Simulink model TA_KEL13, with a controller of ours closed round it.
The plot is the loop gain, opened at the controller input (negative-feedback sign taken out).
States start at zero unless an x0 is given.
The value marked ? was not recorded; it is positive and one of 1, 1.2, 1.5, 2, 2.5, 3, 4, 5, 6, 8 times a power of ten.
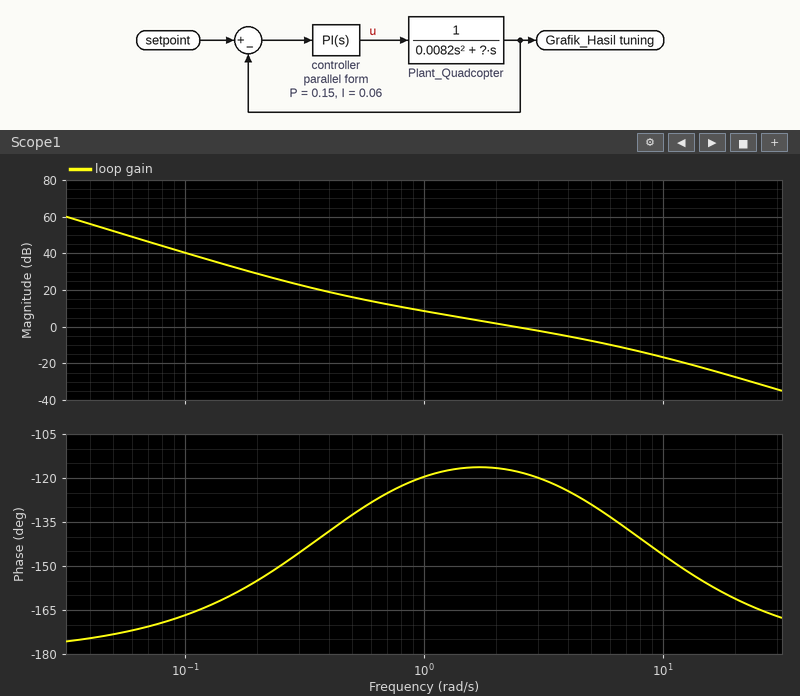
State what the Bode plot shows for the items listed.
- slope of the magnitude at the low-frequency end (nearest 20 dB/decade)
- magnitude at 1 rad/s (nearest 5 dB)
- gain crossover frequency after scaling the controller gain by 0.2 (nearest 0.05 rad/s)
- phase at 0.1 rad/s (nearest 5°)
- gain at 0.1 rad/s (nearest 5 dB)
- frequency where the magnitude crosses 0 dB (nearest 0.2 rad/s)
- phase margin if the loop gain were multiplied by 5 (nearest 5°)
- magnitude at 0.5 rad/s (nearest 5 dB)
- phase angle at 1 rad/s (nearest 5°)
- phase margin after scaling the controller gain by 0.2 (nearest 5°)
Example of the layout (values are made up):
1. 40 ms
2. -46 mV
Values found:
1. -40 dB/decade
2. 10 dB
3. 0.60 rad/s
4. -165°
5. 40 dB
6. 2.4 rad/s
7. 40°
8. 15 dB
9. -120°
10. 50°
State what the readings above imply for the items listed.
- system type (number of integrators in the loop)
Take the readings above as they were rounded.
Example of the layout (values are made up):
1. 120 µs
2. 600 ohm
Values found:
1. 2
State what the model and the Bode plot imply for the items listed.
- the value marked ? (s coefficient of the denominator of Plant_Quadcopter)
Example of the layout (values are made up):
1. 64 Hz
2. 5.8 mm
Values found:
1. 0.06
